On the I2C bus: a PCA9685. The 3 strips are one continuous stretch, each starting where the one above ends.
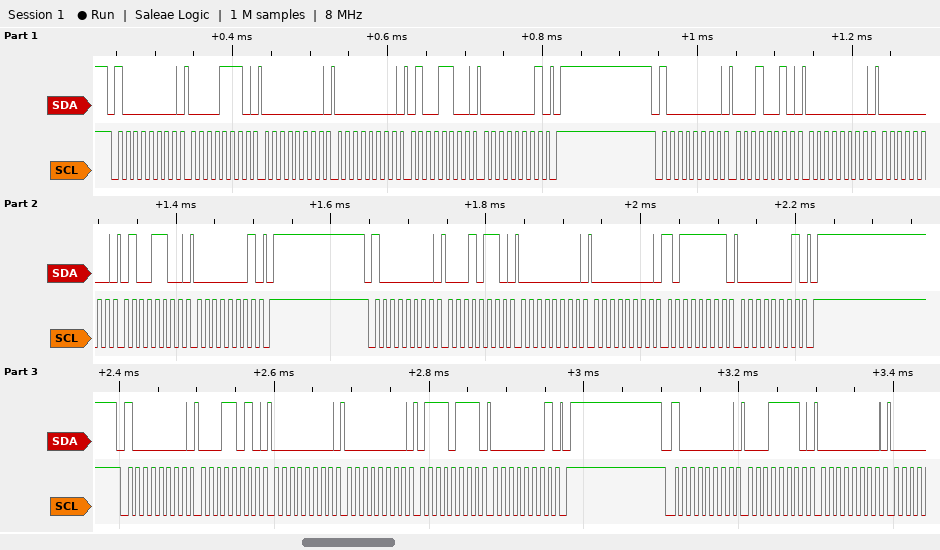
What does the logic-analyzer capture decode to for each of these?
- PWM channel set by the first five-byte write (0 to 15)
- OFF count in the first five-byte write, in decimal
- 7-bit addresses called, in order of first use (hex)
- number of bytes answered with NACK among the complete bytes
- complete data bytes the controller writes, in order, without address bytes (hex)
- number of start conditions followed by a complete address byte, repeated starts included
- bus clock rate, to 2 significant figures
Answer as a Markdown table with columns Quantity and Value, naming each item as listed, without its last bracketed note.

| Quantity | Value |
|---|---|
| PWM channel set by the first five-byte write | 2 |
| OFF count in the first five-byte write, in decimal | 332 |
| 7-bit addresses called, in order of first use | 0x40 |
| number of bytes answered with NACK among the complete bytes | 0 |
| complete data bytes the controller writes, in order, without address bytes | 0E 00 00 4C 01 12 00 00 4C 01 16 00 00 BF 01 1A 00 00 77 01 1E 00 |
| number of start conditions followed by a complete address byte, repeated starts included | 5 |
| bus clock rate, to 2 significant figures | 100 kHz |
